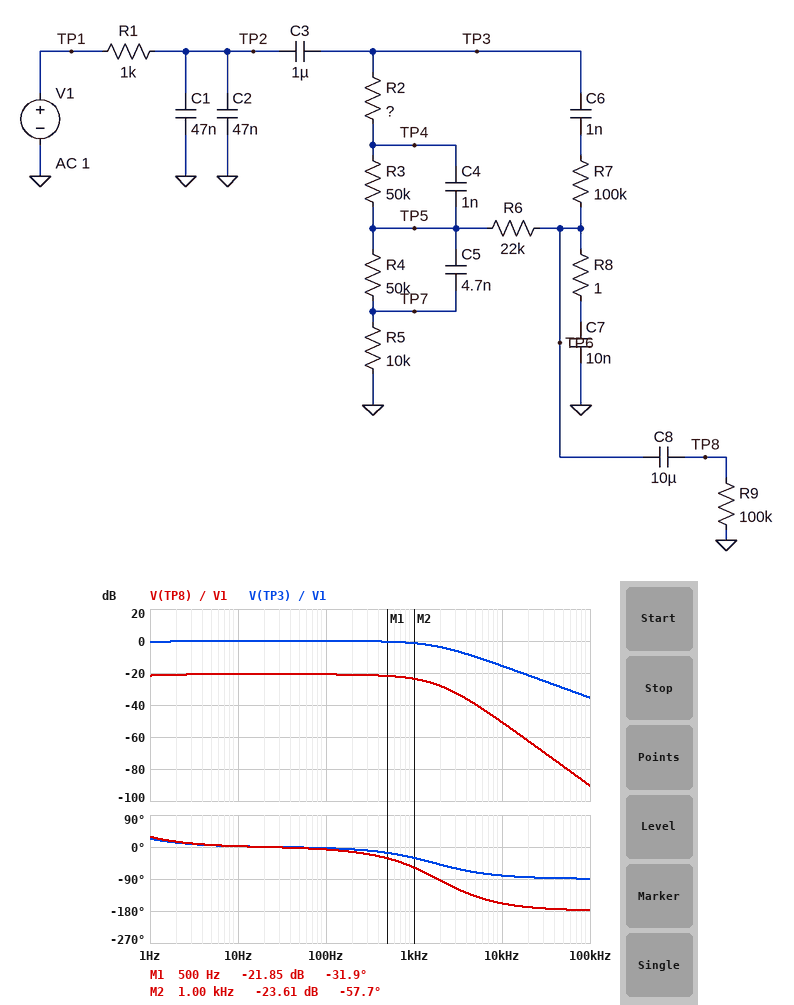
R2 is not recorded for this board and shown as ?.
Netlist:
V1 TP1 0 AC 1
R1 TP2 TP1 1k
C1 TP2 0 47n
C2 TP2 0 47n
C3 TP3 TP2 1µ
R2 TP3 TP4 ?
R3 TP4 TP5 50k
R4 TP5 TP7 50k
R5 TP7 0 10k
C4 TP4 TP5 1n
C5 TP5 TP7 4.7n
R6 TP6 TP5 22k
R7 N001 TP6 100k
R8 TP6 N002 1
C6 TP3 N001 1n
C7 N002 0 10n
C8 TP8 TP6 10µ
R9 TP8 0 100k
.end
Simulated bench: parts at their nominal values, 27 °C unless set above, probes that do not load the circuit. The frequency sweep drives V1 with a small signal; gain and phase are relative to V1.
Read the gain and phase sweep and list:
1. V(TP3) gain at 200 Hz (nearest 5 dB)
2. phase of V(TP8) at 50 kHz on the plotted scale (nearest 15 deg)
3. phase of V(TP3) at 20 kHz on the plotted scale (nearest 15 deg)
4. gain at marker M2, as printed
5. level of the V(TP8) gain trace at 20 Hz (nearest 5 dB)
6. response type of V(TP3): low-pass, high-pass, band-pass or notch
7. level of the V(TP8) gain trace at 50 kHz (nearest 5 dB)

0 dB
-180 deg
-90 deg
-23.61 dB
-20 dB
low-pass
-80 dB
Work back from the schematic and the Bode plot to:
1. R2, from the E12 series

270 kΩ
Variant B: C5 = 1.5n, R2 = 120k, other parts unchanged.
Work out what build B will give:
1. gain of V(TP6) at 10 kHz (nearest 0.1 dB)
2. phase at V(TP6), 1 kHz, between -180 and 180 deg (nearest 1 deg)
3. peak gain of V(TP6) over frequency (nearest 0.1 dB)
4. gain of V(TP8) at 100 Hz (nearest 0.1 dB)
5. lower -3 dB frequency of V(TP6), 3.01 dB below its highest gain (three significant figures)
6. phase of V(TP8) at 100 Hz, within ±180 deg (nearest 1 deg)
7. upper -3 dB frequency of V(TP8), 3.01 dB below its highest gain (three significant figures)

-49.4 dB
-65 deg
-16.2 dB
-16.3 dB
736 mHz
-10 deg
661 Hz
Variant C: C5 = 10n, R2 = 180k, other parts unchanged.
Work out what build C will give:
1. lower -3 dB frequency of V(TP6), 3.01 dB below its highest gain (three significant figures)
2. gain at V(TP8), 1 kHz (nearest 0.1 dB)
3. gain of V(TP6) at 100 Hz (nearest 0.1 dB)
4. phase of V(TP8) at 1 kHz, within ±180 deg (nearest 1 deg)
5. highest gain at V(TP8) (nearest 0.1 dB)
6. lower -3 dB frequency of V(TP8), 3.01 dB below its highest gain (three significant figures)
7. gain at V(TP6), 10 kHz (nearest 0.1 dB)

561 mHz
-24.0 dB
-18.8 dB
-57 deg
-18.3 dB
603 mHz
-50.4 dB
